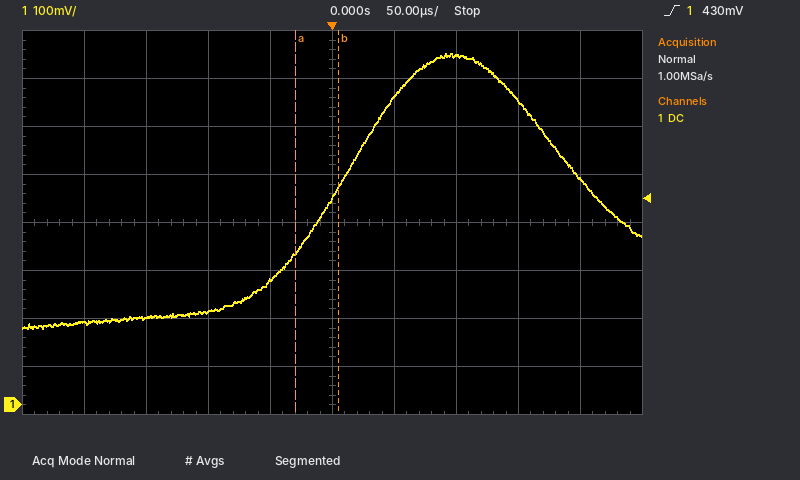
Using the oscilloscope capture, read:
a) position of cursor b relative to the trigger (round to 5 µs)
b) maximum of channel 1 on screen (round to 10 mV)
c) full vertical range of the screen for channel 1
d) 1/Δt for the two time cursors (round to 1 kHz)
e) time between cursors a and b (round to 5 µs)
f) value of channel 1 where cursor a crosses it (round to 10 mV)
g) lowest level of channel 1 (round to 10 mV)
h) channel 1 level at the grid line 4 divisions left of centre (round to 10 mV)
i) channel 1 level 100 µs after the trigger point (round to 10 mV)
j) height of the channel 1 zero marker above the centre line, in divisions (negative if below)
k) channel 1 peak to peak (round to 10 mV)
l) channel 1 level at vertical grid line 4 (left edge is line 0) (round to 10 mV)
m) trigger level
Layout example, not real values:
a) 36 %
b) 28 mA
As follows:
a) +5 µs
b) 730 mV
c) 800 mV
d) 29 kHz
e) 35 µs
f) 320 mV
g) 160 mV
h) 170 mV
i) 730 mV
j) -3.8 div
k) 570 mV
l) 260 mV
m) 430 mV
